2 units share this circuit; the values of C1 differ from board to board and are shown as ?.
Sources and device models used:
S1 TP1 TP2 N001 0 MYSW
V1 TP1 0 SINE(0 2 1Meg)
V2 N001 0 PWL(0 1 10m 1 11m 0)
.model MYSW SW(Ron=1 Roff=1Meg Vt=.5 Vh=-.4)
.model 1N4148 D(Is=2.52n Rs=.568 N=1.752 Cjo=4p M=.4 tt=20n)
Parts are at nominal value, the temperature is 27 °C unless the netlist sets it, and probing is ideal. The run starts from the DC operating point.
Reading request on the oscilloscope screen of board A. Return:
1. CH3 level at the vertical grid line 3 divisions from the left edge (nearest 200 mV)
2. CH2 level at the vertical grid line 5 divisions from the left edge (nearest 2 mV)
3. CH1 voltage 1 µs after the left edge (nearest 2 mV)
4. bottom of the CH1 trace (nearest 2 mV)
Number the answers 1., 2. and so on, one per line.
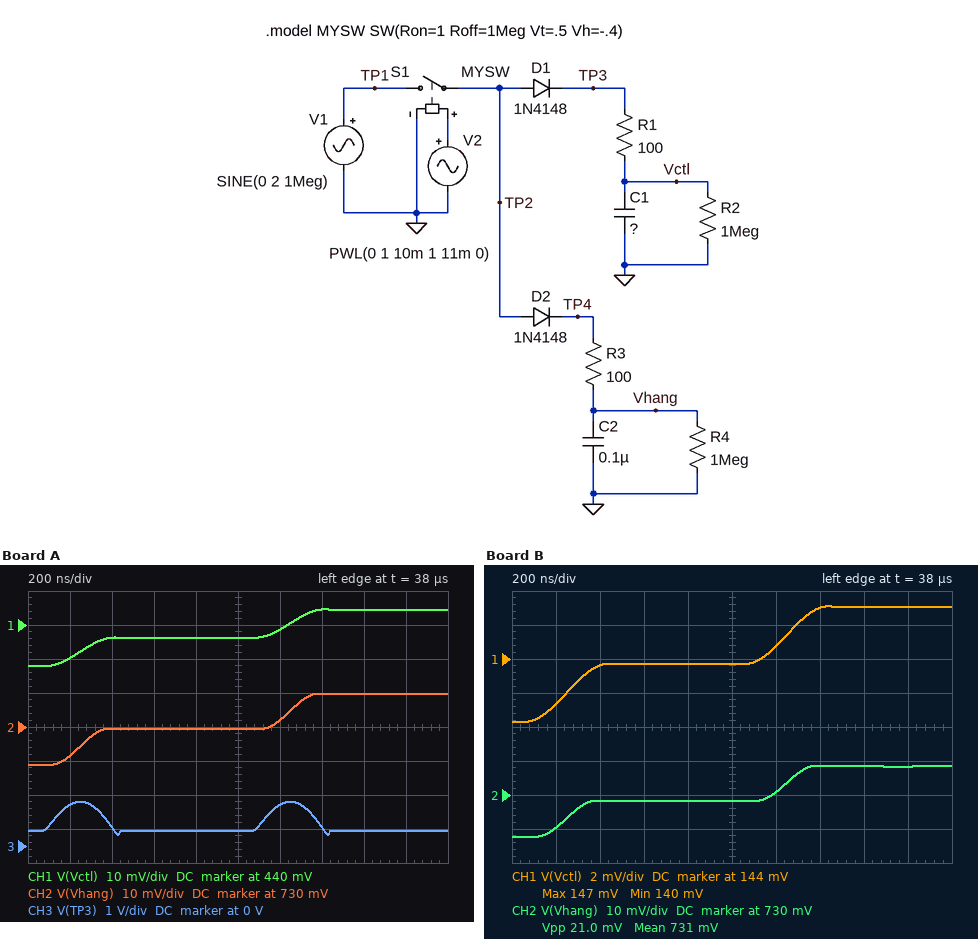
1. 400 mV
2. 730 mV
3. 436 mV
4. 428 mV
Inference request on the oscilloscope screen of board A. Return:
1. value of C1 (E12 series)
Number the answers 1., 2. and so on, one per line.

1. 220 nF
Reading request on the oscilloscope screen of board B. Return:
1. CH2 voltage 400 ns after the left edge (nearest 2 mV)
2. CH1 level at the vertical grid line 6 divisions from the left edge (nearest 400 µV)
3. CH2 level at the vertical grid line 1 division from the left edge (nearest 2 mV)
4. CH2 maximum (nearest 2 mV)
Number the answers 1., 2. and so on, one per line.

1. 728 mV
2. 144.8 mV
3. 720 mV
4. 738 mV
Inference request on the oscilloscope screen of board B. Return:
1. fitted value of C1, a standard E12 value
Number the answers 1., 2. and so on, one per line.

1. 820 nF
